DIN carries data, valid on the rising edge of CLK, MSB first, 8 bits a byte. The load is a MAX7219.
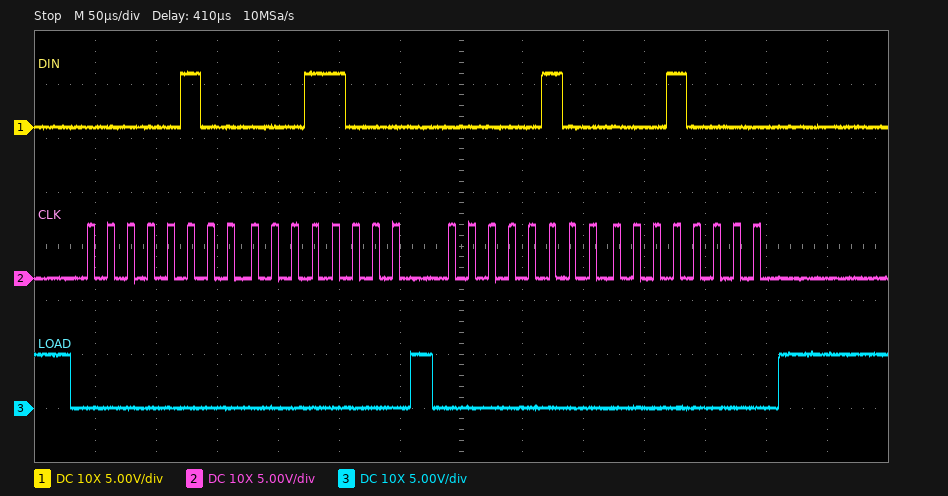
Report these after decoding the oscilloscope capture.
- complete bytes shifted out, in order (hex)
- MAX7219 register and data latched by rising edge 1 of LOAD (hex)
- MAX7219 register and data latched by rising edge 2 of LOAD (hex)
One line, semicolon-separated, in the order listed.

04 18 04 10; register 0x4, data 0x18; register 0x4, data 0x10
